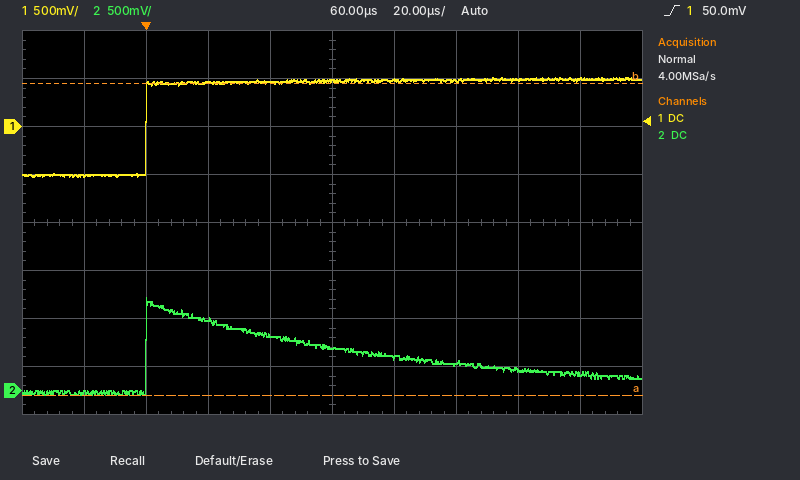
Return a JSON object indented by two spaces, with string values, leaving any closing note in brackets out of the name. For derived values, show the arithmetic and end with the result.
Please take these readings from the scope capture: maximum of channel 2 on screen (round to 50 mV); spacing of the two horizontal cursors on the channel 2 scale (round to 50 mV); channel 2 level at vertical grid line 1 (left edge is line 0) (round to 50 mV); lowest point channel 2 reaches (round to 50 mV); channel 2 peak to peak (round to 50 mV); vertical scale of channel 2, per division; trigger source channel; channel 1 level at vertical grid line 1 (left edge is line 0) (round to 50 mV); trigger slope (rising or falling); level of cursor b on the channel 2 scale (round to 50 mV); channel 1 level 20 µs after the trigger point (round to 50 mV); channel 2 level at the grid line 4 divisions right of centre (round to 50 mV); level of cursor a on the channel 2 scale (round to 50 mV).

{
  "maximum of channel 2 on screen": "950 mV",
  "spacing of the two horizontal cursors on the channel 2 scale": "3.25 V",
  "channel 2 level at vertical grid line 1 (left edge is line 0)": "0 mV",
  "lowest point channel 2 reaches": "-50 mV",
  "channel 2 peak to peak": "950 mV − (-50 mV) = 1.00 V",
  "vertical scale of channel 2, per division": "500 mV",
  "trigger source channel": "channel 1",
  "channel 1 level at vertical grid line 1 (left edge is line 0)": "-500 mV",
  "trigger slope": "rising",
  "level of cursor b on the channel 2 scale": "3.20 V",
  "channel 1 level 20 µs after the trigger point": "450 mV",
  "channel 2 level at the grid line 4 divisions right of centre": "200 mV",
  "level of cursor a on the channel 2 scale": "-50 mV"
}
